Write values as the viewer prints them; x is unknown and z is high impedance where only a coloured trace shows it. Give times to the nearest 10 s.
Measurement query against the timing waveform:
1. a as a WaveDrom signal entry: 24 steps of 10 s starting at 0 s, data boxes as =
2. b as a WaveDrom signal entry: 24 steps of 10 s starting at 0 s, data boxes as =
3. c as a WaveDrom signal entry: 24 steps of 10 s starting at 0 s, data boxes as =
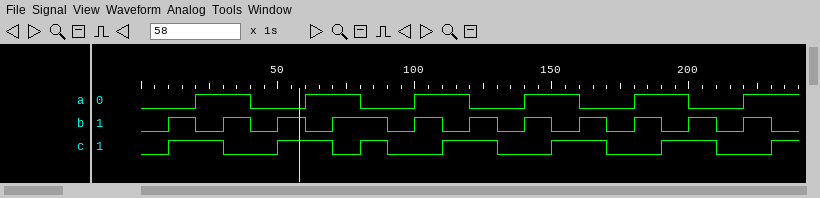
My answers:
{name: 'a', wave: '0.1.0.1.0.1.0.1.0.1.0.1.'}
{name: 'b', wave: '01010101.010101010101010'}
{name: 'c', wave: '01.0.1.010.1.0.1.0.1.0.1'}
